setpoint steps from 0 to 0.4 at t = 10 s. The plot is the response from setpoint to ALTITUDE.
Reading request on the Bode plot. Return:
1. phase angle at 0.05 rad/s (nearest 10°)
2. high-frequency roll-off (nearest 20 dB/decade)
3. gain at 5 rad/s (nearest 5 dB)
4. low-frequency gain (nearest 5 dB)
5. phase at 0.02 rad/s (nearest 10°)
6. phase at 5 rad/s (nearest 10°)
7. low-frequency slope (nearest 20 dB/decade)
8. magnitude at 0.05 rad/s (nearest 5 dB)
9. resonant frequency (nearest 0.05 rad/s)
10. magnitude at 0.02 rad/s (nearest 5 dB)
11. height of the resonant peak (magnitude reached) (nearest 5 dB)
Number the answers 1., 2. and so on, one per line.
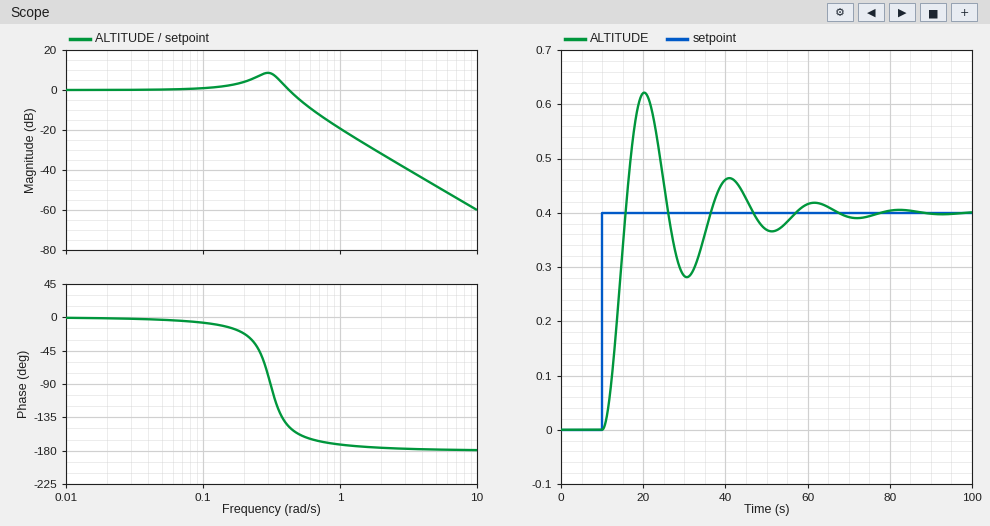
1. 0°
2. -40 dB/decade
3. -50 dB
4. 0 dB
5. 0°
6. -180°
7. 0 dB/decade
8. 0 dB
9. 0.30 rad/s
10. 0 dB
11. 10 dB
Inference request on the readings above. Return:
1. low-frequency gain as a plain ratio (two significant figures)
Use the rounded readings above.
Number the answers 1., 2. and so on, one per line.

1. 1.0
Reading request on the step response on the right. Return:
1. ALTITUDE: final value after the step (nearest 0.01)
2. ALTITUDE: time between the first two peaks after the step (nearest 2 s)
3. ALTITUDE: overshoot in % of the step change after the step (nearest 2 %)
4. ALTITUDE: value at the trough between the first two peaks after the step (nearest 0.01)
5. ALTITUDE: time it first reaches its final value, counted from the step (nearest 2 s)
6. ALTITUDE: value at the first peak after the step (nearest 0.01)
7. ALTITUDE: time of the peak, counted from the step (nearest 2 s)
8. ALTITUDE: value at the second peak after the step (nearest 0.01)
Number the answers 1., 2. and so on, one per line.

1. 0.40
2. 20 s
3. 56 %
4. 0.28
5. 6 s
6. 0.62
7. 10 s
8. 0.46
